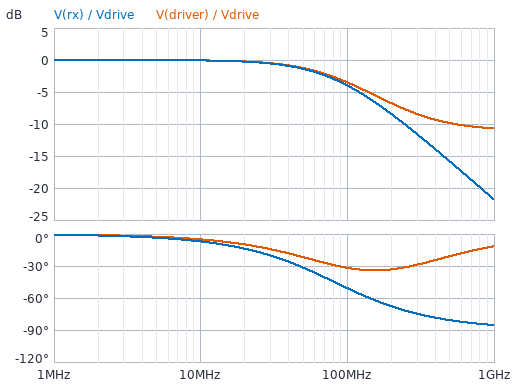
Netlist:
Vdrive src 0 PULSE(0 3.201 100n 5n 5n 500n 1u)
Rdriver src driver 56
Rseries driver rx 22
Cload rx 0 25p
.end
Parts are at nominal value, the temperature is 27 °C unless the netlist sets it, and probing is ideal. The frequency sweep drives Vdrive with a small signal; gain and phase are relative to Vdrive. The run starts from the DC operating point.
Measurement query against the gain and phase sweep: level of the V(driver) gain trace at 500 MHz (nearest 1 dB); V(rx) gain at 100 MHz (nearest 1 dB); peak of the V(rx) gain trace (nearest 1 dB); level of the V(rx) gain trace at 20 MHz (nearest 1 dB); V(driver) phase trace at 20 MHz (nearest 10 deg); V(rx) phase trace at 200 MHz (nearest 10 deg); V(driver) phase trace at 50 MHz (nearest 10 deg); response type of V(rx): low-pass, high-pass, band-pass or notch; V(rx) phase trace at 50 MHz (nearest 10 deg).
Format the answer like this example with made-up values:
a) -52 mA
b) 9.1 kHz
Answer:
a) -10 dB
b) -4 dB
c) 0 dB
d) 0 dB
e) -10 deg
f) -70 deg
g) -20 deg
h) low-pass
i) -30 deg
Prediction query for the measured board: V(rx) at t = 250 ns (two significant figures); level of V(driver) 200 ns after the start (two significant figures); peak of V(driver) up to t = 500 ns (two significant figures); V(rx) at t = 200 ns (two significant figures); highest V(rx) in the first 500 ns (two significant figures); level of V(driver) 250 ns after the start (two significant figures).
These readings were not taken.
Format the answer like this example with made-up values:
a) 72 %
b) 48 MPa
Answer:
a) 3.2 V
b) 3.2 V
c) 3.2 V
d) 3.2 V
e) 3.2 V
f) 3.2 V
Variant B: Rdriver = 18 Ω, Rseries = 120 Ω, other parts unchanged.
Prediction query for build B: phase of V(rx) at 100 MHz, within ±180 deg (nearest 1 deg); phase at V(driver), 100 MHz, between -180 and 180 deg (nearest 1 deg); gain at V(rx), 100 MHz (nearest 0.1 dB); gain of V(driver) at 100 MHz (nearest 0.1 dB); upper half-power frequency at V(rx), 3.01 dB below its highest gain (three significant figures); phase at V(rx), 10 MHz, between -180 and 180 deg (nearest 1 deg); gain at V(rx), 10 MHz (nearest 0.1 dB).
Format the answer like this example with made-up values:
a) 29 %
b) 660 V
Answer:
a) -65 deg
b) -3 deg
c) -7.6 dB
d) -1.0 dB
e) 46.1 MHz
f) -12 deg
g) -0.2 dB
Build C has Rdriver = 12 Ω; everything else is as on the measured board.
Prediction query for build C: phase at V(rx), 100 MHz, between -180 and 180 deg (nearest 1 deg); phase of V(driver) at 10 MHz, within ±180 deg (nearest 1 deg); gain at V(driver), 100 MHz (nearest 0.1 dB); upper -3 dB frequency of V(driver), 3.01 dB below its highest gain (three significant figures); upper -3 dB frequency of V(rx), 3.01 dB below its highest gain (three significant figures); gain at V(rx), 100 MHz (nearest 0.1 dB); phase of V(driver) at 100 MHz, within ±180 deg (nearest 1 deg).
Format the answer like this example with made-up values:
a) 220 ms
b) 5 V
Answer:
a) -28 deg
b) -1 deg
c) -0.6 dB
d) 464 MHz
e) 187 MHz
f) -1.1 dB
g) -9 deg
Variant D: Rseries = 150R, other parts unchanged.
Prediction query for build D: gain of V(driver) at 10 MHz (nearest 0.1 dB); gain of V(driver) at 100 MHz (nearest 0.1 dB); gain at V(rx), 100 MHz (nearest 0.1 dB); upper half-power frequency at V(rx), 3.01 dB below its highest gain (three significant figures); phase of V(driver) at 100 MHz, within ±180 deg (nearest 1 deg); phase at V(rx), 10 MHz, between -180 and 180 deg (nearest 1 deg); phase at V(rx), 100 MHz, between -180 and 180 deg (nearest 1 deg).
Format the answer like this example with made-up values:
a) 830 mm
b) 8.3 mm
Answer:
a) -0.2 dB
b) -2.4 dB
c) -10.6 dB
d) 30.9 MHz
e) -6 deg
f) -18 deg
g) -73 deg
